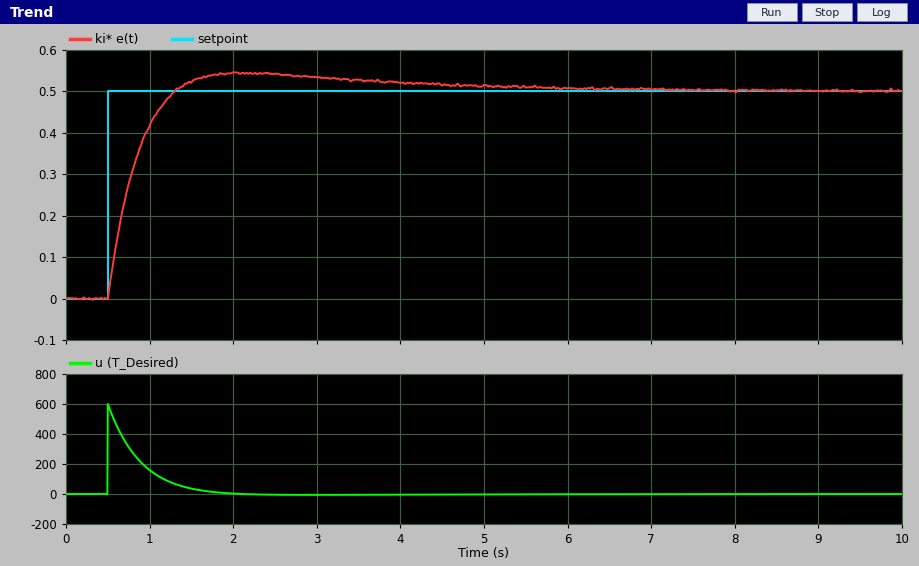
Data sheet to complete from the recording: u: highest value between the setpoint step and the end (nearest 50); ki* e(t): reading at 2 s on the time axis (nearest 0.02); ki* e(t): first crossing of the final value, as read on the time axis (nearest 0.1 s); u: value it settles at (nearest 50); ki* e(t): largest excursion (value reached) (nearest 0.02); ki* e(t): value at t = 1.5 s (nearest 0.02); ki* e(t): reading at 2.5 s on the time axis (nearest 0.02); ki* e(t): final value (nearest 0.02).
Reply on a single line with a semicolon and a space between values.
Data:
600; 0.54; 1.3 s; 0; 0.54; 0.52; 0.54; 0.50
